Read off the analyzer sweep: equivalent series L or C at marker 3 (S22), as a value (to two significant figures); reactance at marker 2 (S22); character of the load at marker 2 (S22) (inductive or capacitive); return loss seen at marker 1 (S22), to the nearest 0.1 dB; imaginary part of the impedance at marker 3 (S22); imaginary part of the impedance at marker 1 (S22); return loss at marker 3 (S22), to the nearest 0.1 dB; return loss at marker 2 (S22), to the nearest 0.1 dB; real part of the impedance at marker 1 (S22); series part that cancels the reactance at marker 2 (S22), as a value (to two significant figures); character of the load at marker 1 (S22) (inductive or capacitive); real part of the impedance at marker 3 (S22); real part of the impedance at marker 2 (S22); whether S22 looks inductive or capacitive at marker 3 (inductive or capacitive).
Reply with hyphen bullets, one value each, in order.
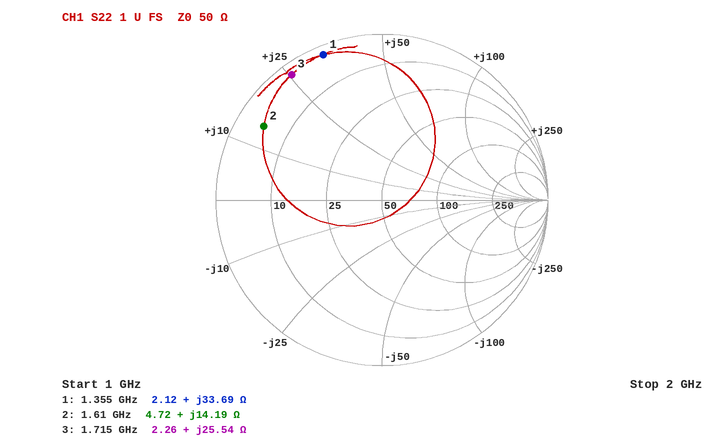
- 2.4 nH
- +14.19 Ω
- inductive
- 0.5 dB
- +25.54 Ω
- +33.69 Ω
- 0.6 dB
- 1.5 dB
- 2.12 Ω
- 7.0 pF
- inductive
- 2.26 Ω
- 4.72 Ω
- inductive
